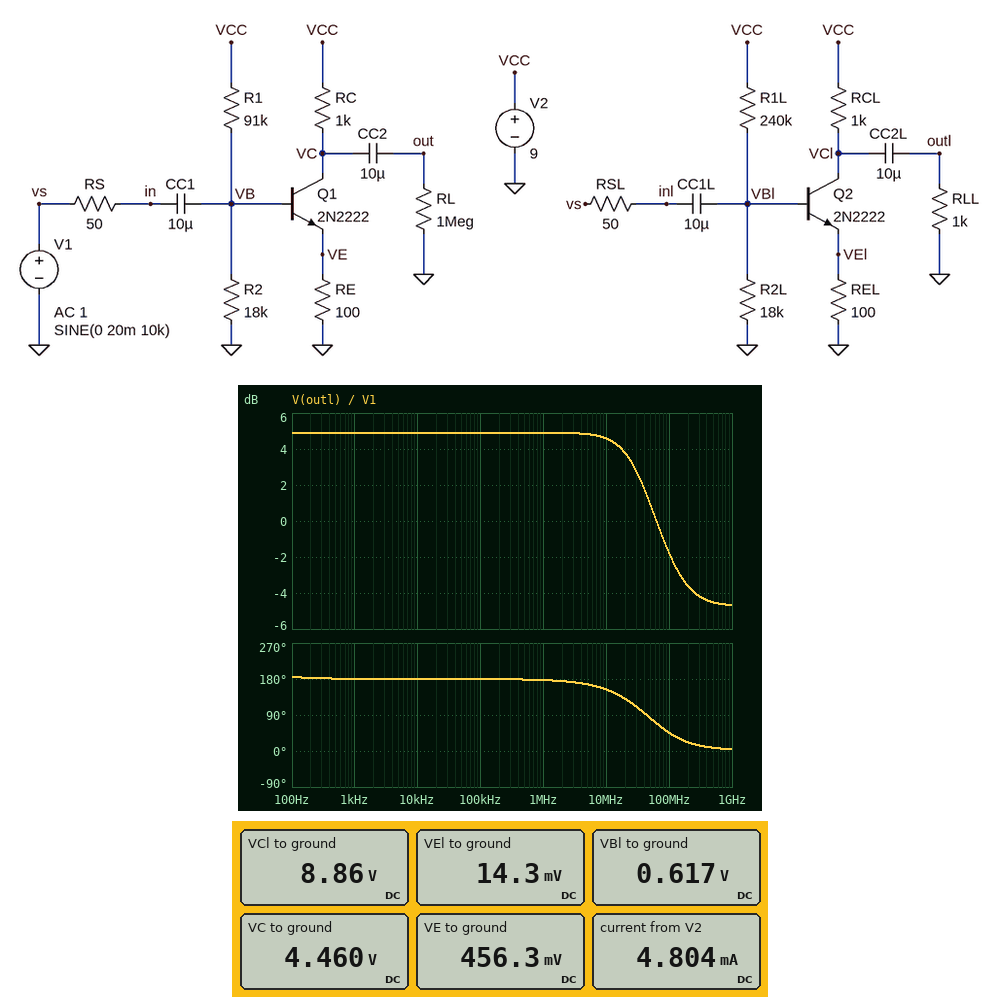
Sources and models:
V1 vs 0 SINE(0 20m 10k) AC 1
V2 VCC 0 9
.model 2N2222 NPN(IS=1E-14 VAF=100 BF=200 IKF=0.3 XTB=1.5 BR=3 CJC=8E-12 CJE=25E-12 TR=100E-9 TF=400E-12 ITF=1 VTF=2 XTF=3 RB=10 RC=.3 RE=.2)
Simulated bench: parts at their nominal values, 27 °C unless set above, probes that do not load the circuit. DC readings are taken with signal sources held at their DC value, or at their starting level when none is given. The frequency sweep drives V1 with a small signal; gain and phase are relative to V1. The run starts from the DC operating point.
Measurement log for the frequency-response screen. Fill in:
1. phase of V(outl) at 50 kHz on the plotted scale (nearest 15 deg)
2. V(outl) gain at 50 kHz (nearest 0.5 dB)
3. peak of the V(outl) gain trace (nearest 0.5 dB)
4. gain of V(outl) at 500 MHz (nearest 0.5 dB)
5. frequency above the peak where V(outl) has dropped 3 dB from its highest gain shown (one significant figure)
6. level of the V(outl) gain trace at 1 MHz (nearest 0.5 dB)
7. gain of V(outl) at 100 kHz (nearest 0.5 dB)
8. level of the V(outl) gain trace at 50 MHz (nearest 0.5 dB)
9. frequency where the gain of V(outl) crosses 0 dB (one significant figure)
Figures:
180 deg
5.0 dB
5.0 dB
-4.5 dB
40 MHz
5.0 dB
5.0 dB
1.0 dB
60 MHz
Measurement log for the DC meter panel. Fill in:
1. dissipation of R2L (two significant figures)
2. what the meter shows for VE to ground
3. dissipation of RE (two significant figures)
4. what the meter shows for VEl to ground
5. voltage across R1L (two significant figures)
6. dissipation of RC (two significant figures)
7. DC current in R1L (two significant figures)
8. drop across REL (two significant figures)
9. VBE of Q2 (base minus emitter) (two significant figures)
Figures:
21 µW
456.3 mV
2.1 mW
14.3 mV
8.4 V
21 mW
35 µA
14 mV
600 mV
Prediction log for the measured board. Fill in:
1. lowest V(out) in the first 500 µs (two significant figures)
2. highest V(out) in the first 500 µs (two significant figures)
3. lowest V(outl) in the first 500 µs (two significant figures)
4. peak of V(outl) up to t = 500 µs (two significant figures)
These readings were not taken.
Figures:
-190 mV
190 mV
-41 mV
30 mV
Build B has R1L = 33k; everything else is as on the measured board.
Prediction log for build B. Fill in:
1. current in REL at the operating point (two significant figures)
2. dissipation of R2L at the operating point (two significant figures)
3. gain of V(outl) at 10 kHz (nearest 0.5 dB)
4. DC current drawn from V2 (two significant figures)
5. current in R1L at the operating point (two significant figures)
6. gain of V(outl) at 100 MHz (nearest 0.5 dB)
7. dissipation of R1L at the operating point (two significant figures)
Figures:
8.2 mA
130 µW
-4.0 dB
13 mA
230 µA
-4.5 dB
1.7 mW
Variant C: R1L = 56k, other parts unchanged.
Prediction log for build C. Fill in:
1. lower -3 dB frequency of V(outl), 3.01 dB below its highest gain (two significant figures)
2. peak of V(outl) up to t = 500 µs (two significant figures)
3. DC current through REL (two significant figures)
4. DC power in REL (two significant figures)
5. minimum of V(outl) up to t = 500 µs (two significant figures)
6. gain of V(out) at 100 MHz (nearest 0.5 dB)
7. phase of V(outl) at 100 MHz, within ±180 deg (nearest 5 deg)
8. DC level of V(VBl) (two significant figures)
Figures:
24 Hz
92 mV
8.1 mA
6.5 mW
-42 mV
6.0 dB
10 deg
1.5 V
